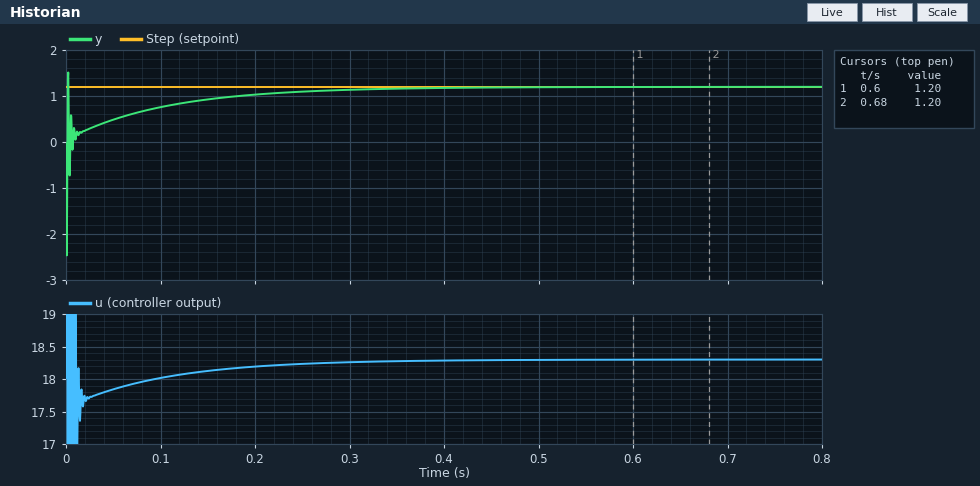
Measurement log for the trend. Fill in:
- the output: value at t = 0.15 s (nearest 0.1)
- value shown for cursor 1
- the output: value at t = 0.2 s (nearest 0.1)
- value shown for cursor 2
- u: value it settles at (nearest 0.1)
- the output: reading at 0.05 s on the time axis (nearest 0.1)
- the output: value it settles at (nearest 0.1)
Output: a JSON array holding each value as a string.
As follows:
["0.9", "1.20", "1.0", "1.20", "18.3", "0.5", "1.2"]
